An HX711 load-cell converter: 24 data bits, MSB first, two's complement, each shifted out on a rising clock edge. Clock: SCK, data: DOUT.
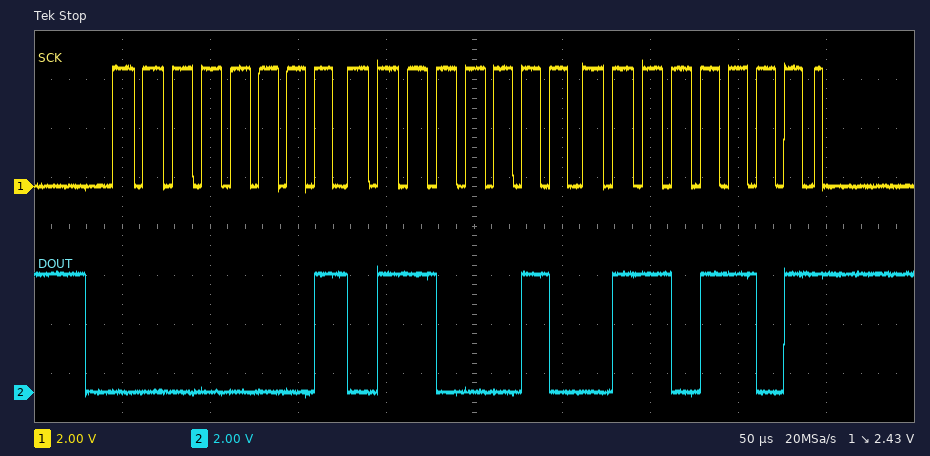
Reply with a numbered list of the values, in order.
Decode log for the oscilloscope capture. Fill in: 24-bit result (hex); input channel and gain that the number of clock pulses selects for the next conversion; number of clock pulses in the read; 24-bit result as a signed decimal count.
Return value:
1. 0x01626D
2. channel A, gain 128
3. 25
4. 90733
